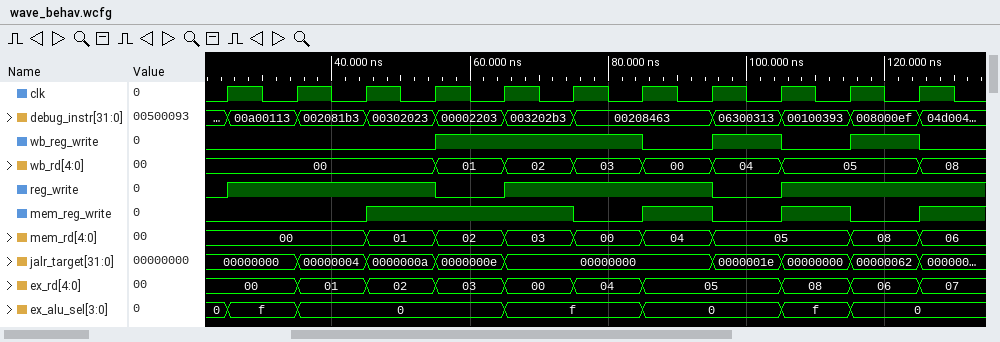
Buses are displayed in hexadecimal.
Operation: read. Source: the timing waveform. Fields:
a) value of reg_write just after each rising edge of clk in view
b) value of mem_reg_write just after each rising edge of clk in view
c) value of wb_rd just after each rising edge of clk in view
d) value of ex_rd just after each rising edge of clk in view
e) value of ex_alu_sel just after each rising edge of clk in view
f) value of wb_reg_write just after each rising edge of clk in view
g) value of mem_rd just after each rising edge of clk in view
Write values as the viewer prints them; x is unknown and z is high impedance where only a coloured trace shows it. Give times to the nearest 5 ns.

1 1 1 0 1 1 1 0 1 1 1
0 0 1 1 1 0 1 0 1 0 1
00, 00, 00, 01, 02, 03, 00, 04, 05, 05, 08
00, 01, 02, 03, 00, 04, 05, 05, 08, 06, 07
f, 0, 0, 0, f, f, 0, 0, f, 0, 0
0 0 0 1 1 1 0 1 0 1 0
00, 00, 01, 02, 03, 00, 04, 05, 05, 08, 06
